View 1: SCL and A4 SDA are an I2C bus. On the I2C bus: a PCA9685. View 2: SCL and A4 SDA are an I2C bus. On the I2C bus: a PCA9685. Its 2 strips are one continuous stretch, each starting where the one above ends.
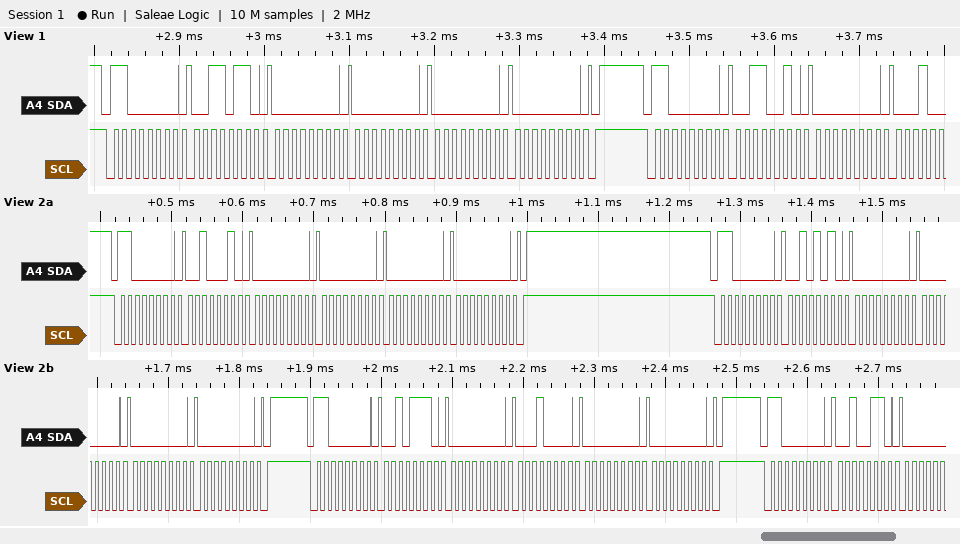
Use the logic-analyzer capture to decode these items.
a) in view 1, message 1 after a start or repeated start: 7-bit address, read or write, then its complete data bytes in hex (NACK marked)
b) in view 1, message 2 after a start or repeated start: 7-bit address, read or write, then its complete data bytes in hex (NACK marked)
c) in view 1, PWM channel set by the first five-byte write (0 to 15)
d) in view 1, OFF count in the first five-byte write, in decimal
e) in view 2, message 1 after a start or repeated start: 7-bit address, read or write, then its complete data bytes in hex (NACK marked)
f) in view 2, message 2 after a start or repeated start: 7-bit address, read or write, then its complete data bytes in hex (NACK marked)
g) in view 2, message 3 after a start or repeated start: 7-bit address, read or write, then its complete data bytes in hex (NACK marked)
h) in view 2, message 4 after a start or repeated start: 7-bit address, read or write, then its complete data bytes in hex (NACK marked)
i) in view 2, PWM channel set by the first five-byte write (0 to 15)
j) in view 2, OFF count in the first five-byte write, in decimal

0x60 write: 36 00 00 00 00
0x60 write: 32 00
12
0
0x60 write: 22 00 00 00 00
0x60 write: 2A 00 00 00 00
0x60 write: 2E 00 10 00 00
0x60 write: 26
7
0
